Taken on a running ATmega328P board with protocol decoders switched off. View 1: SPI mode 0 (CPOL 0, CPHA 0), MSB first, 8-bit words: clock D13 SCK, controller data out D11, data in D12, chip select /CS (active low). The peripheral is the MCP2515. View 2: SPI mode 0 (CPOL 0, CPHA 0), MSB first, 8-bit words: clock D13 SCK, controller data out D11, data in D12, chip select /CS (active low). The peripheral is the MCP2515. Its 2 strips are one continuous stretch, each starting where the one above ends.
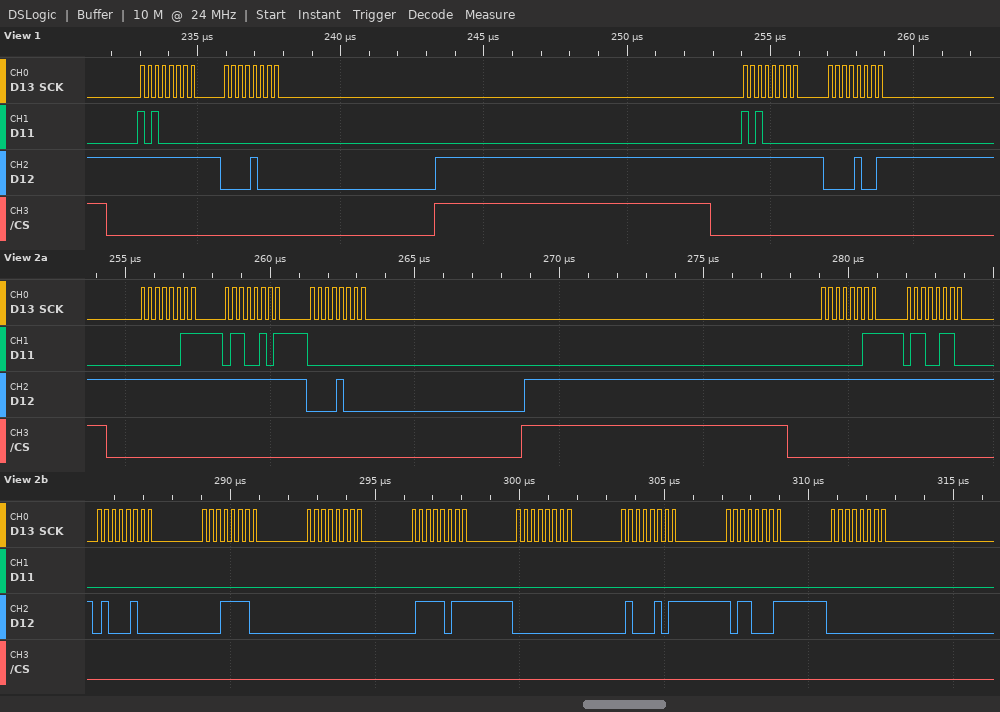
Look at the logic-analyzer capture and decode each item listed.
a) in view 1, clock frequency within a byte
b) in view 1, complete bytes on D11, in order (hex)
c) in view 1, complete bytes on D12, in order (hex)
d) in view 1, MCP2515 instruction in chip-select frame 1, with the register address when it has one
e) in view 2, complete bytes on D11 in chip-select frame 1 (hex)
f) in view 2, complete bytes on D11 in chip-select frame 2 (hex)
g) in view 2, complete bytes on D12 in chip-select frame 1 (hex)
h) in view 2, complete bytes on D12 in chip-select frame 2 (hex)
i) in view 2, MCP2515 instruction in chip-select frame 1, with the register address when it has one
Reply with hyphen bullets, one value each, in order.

- 4 MHz
- A0 00 A0 00
- FF 08 FF 09
- READ STATUS
- 03 65 00
- 03 66 00 00 00 00 00 00 00 00
- FF FF 08
- FF FF 44 1E 00 7B 00 45 B1 00
- READ 0x65
